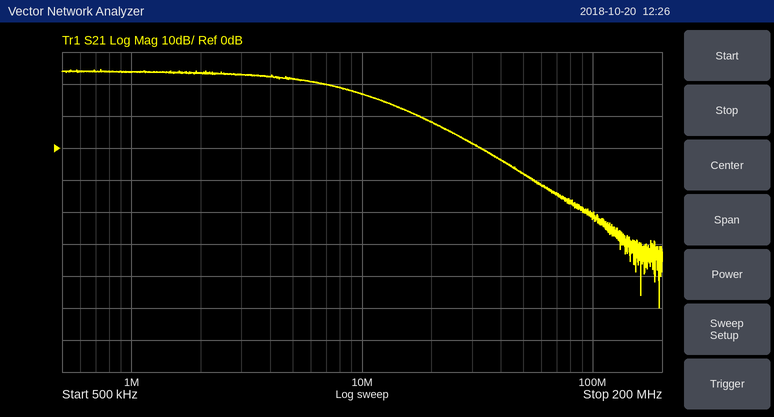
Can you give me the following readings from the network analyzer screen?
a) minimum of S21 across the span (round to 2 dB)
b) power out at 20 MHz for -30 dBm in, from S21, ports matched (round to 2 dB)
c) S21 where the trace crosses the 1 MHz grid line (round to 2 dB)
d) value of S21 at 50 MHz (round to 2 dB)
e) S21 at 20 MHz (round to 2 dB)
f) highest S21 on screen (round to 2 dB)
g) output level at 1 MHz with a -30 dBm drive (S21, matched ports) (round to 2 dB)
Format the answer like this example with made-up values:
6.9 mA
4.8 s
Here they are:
-50 dB
-22 dBm
24 dB
-8 dB
8 dB
24 dB
-6 dBm
